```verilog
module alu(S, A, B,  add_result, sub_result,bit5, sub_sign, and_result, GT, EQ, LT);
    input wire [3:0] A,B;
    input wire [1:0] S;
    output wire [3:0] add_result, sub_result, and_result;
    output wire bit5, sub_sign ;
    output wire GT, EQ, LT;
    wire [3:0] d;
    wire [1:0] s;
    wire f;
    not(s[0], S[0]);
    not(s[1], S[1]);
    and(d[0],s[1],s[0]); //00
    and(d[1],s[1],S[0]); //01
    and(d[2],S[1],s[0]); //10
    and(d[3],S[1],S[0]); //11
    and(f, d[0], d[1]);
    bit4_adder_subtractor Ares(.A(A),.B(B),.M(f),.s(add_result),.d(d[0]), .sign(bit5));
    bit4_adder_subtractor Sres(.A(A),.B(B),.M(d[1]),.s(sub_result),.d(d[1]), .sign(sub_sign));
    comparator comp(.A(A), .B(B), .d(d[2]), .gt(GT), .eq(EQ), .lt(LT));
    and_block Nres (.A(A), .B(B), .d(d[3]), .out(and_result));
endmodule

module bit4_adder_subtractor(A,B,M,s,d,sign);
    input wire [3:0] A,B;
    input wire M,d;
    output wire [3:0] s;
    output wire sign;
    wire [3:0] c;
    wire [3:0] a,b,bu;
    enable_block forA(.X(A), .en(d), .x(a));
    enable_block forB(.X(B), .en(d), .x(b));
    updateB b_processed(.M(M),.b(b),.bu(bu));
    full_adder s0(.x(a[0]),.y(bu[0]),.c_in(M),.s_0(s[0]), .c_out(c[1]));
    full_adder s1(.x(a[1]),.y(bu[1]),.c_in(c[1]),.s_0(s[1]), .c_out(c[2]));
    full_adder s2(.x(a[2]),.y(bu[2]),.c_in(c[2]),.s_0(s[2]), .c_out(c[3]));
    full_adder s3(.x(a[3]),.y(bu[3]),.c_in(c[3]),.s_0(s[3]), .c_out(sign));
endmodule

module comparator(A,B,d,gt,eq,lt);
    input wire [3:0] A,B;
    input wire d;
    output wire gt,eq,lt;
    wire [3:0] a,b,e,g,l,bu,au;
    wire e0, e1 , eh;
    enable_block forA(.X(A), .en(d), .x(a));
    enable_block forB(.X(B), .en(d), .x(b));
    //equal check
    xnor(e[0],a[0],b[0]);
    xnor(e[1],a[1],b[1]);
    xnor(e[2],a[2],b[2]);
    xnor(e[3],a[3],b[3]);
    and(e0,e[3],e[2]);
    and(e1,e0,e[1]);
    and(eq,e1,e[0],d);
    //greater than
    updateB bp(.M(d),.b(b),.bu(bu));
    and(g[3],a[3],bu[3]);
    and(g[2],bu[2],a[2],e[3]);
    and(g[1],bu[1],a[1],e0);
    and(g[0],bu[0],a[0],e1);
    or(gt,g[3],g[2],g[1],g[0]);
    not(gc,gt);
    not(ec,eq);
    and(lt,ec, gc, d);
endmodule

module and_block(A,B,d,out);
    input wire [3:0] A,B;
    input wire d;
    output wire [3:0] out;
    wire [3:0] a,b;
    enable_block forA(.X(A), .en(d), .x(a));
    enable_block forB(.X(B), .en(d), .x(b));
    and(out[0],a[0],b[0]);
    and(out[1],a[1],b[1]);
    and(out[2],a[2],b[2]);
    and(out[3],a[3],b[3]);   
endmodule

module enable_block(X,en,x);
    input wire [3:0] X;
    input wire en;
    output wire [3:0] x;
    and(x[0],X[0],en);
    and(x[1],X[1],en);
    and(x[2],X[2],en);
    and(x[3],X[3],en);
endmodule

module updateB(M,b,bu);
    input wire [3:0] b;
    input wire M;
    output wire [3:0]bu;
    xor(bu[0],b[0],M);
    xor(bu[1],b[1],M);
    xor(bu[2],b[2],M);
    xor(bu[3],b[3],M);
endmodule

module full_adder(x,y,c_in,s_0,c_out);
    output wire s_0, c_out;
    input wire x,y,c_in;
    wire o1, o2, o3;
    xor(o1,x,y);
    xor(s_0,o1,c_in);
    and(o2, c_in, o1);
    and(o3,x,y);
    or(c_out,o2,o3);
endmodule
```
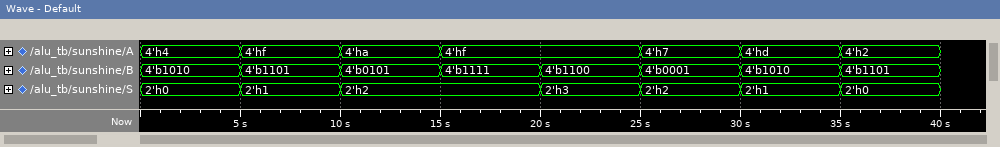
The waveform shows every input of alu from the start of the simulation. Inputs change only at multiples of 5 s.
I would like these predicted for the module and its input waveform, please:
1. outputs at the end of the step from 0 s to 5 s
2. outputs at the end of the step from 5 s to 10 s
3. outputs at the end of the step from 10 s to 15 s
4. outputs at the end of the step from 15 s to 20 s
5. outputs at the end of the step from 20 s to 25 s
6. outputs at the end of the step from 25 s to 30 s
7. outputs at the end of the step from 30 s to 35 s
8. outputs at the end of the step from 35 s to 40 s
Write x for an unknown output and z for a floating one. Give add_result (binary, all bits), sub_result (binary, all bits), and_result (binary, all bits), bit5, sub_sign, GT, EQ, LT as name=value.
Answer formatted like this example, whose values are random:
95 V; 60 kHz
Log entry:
add_result=1110, sub_result=0000, and_result=0000, bit5=0, sub_sign=0, GT=0, EQ=0, LT=0; add_result=0000, sub_result=0010, and_result=0000, bit5=0, sub_sign=1, GT=0, EQ=0, LT=0; add_result=0000, sub_result=0000, and_result=0000, bit5=0, sub_sign=0, GT=1, EQ=0, LT=0; add_result=0000, sub_result=0000, and_result=0000, bit5=0, sub_sign=0, GT=0, EQ=1, LT=0; add_result=0000, sub_result=0000, and_result=1100, bit5=0, sub_sign=0, GT=0, EQ=0, LT=0; add_result=0000, sub_result=0000, and_result=0000, bit5=0, sub_sign=0, GT=1, EQ=0, LT=0; add_result=0000, sub_result=0011, and_result=0000, bit5=0, sub_sign=1, GT=0, EQ=0, LT=0; add_result=1111, sub_result=0000, and_result=0000, bit5=0, sub_sign=0, GT=0, EQ=0, LT=0
